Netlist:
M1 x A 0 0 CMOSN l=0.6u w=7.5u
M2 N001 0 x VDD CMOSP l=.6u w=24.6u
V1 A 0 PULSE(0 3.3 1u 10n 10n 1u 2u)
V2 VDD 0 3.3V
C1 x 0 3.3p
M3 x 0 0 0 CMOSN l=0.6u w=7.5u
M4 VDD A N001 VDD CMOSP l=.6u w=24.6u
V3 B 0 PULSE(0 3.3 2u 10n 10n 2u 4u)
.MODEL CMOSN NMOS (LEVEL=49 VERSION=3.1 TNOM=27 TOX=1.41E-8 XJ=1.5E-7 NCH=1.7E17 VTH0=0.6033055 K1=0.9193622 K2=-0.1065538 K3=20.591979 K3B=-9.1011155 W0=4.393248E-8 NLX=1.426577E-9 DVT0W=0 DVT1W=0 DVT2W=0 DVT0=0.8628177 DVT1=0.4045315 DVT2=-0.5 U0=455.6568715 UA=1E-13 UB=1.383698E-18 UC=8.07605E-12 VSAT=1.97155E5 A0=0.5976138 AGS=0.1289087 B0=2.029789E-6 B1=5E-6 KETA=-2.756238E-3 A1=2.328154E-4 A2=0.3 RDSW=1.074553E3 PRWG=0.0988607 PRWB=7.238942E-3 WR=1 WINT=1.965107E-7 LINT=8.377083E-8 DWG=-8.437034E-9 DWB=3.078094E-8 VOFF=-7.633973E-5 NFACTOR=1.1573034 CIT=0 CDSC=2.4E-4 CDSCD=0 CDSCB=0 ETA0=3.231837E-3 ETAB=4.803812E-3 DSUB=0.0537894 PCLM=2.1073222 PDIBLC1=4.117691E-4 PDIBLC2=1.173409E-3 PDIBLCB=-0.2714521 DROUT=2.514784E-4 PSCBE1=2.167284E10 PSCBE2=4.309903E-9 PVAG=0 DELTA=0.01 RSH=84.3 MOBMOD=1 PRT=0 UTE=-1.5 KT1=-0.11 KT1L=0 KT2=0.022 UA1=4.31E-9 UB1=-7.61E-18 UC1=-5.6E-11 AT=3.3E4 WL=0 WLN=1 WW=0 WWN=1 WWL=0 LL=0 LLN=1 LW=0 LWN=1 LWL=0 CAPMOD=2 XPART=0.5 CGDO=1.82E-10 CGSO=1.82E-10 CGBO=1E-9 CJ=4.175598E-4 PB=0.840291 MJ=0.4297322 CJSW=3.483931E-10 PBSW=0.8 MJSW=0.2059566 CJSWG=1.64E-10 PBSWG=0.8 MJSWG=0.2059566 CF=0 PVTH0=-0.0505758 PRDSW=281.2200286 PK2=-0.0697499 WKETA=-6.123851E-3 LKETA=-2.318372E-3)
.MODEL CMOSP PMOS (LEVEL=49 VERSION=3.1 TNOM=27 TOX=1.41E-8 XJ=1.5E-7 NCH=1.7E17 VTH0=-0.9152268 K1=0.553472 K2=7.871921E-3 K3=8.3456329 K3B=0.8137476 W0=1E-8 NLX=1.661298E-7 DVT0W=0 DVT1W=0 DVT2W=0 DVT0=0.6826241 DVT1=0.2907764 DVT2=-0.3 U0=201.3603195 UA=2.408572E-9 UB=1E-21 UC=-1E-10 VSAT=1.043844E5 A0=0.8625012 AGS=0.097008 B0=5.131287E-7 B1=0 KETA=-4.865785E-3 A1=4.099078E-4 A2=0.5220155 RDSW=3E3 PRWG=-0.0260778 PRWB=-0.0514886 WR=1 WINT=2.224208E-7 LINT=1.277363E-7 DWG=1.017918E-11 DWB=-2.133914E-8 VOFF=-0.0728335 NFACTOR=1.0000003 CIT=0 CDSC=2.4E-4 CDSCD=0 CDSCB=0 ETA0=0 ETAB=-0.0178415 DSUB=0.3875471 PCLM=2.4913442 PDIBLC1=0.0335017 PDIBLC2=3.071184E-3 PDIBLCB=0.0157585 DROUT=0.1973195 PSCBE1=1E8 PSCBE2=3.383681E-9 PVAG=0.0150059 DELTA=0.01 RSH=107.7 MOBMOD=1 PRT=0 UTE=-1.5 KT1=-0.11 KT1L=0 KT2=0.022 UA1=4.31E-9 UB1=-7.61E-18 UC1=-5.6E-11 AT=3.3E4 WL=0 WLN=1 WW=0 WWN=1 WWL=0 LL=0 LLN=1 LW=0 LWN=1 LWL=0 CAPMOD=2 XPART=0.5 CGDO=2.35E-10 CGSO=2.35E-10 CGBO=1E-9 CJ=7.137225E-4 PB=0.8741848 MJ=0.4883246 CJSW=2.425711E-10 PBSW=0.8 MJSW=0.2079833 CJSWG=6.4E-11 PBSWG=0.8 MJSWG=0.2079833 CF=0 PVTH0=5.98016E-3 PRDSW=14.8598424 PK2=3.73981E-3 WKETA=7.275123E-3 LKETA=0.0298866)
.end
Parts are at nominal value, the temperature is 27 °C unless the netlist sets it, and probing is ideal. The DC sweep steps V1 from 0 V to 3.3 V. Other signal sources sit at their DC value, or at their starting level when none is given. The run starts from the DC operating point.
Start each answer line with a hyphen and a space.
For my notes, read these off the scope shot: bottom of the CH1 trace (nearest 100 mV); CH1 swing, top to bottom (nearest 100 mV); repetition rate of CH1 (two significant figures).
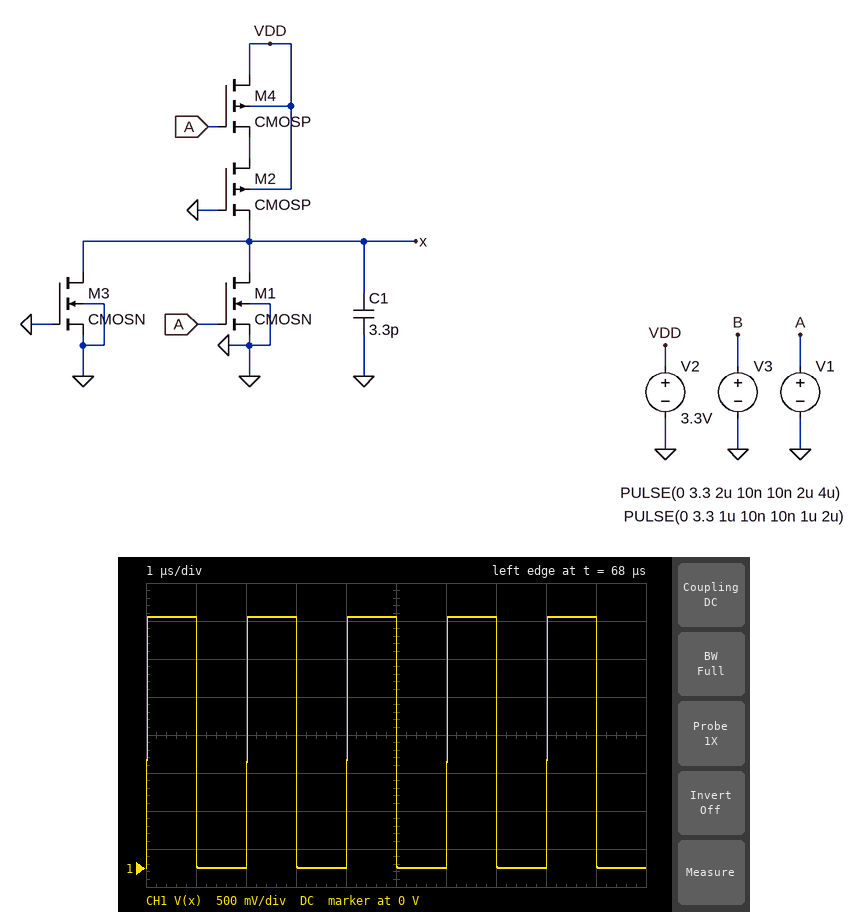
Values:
- 0 V
- 3.3 V
- 500 kHz
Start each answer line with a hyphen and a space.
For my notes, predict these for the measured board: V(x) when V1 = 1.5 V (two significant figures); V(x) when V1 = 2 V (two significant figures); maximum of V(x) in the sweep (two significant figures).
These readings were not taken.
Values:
- 2.4 V
- 140 mV
- 3.3 V
